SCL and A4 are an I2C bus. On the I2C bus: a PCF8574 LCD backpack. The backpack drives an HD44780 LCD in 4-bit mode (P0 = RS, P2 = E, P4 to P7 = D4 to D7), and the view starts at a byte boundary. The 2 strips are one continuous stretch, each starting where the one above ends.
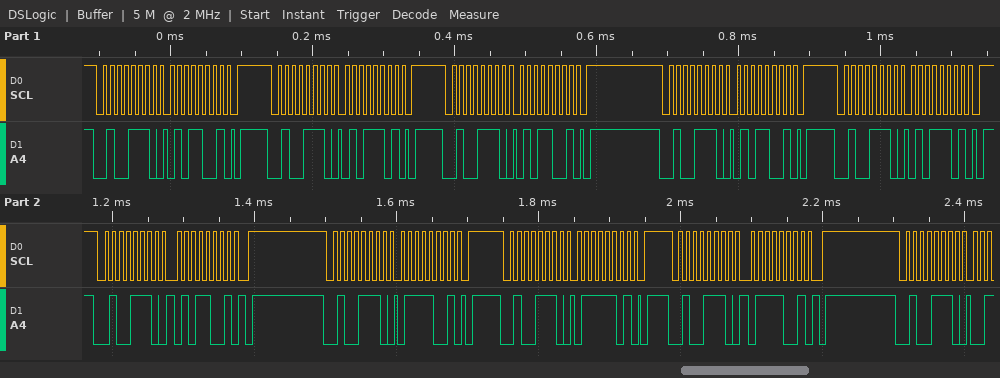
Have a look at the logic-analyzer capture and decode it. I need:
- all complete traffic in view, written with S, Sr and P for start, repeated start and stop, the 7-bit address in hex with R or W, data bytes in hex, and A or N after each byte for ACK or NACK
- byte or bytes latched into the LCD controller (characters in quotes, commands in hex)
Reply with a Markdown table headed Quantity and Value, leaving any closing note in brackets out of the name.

| Quantity | Value |
|---|---|
| all complete traffic in view, written with S, Sr and P for start, repeated start and stop, the 7-bit address in hex with R or W, data bytes in hex, and A or N after each byte for ACK or NACK | S 27W A 59 A P S 27W A 5D A P S 27W A 59 A P S 27W A 59 A P S 27W A 5D A P S 27W A 59 A P S 27W A 79 A P S 27W A 7D A P S 27W A 79 A P S 27W A |
| byte or bytes latched into the LCD controller | 'U' |
